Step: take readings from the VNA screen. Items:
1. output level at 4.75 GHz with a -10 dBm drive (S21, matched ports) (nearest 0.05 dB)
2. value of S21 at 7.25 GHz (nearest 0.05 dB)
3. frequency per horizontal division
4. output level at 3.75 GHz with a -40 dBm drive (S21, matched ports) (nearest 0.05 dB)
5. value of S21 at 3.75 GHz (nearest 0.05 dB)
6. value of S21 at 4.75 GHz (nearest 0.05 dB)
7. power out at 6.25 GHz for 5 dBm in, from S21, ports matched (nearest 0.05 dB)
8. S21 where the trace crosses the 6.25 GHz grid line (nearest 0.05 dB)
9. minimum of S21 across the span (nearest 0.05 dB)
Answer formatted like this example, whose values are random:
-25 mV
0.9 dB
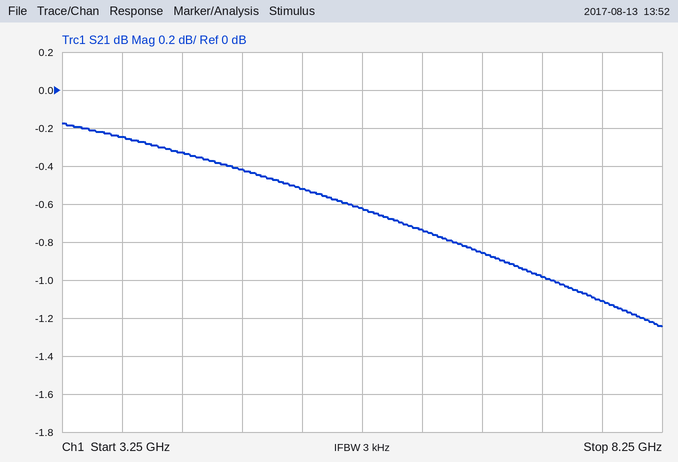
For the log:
-10.40 dBm
-1.00 dB
500 MHz
-40.25 dBm
-0.25 dB
-0.40 dB
4.25 dBm
-0.75 dB
-1.25 dB
